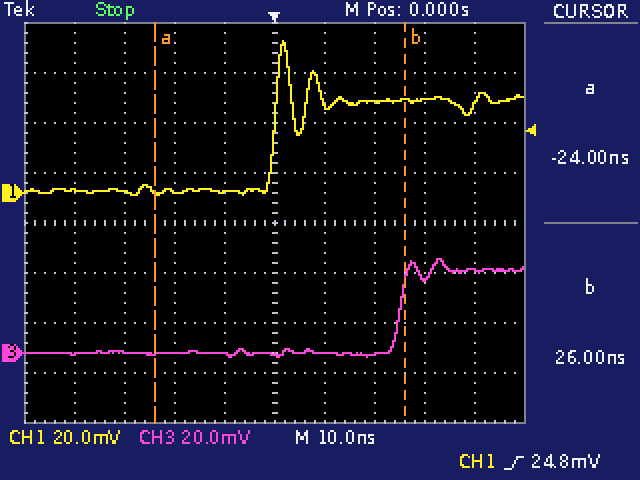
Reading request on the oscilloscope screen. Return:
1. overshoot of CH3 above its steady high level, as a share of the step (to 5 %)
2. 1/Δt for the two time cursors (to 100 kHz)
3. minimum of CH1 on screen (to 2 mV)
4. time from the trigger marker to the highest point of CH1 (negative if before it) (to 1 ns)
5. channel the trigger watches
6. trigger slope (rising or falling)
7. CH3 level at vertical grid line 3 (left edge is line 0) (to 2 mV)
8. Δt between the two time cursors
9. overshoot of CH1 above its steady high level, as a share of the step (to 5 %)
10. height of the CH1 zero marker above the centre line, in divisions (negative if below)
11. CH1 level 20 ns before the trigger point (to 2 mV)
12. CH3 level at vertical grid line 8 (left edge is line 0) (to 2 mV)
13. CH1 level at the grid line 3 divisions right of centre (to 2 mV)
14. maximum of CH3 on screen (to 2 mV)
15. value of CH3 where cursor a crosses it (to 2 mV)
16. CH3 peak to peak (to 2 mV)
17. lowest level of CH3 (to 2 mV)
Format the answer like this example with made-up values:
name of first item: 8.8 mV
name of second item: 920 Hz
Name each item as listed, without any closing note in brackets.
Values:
overshoot of CH3 above its steady high level, as a share of the step: 15 %
1/Δt for the two time cursors: 20.0 MHz
minimum of CH1 on screen: 0 mV
time from the trigger marker to the highest point of CH1 (negative if before it): +2 ns
channel the trigger watches: CH1
trigger slope: rising
CH3 level at vertical grid line 3 (left edge is line 0): 0 mV
Δt between the two time cursors: 50 ns
overshoot of CH1 above its steady high level, as a share of the step: 65 %
height of the CH1 zero marker above the centre line, in divisions: +0.6 div
CH1 level 20 ns before the trigger point: 0 mV
CH3 level at vertical grid line 8 (left edge is line 0): 30 mV
CH1 level at the grid line 3 divisions right of centre: 38 mV
maximum of CH3 on screen: 38 mV
value of CH3 where cursor a crosses it: 0 mV
CH3 peak to peak: 40 mV
lowest level of CH3: -2 mV
